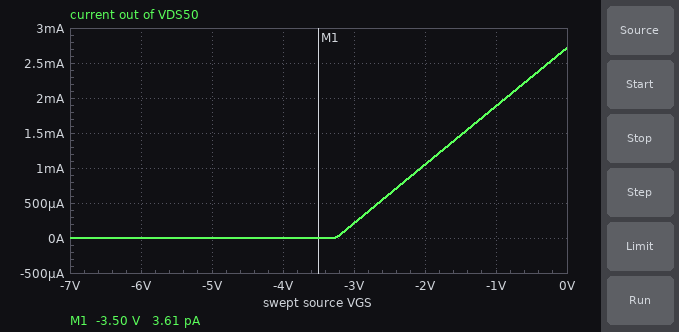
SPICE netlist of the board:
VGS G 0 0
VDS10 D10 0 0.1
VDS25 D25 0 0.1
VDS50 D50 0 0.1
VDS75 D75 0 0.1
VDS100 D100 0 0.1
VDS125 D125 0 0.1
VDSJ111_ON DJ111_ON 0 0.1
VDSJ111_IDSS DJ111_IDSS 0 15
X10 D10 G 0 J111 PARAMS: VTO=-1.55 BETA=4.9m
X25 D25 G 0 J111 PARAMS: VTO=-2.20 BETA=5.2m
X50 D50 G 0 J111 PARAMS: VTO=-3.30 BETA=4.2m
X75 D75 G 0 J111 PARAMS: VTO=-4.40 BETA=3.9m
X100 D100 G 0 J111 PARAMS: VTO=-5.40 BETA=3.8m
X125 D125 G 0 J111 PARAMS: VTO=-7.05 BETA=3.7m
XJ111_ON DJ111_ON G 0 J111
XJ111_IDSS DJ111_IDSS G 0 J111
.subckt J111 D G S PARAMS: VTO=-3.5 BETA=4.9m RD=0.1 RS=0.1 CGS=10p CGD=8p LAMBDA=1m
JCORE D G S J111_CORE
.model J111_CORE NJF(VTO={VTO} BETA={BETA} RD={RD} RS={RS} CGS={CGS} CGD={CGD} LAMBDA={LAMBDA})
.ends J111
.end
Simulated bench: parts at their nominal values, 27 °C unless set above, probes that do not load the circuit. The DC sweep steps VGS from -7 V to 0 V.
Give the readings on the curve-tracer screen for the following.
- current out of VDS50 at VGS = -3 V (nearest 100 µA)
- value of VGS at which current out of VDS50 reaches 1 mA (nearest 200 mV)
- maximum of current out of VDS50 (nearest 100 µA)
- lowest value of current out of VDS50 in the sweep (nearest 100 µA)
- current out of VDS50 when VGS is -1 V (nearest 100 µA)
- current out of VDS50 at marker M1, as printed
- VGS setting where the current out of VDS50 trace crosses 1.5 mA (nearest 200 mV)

200 µA
-2.0 V
2.7 mA
0 A
1.9 mA
3.61 pA
-1.4 V
